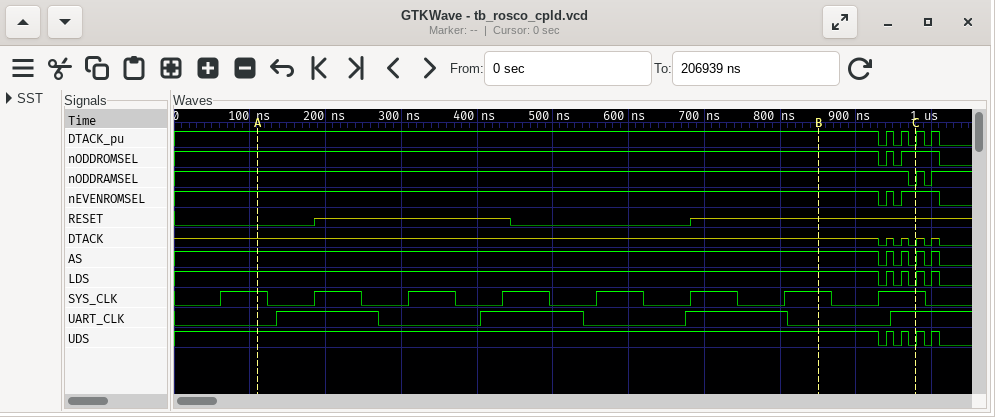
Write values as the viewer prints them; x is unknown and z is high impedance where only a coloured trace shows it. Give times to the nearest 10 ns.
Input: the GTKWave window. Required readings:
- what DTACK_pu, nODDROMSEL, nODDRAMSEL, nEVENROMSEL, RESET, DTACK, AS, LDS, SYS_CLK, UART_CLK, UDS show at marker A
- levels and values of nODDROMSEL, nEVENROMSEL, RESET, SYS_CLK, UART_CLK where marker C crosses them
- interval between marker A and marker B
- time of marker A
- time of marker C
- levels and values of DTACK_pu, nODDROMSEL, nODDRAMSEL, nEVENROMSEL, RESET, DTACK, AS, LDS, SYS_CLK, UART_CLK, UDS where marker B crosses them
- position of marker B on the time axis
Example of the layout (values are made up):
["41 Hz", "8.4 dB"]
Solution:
["DTACK_pu=1, nODDROMSEL=1, nODDRAMSEL=1, nEVENROMSEL=1, RESET=0, DTACK=z, AS=1, LDS=1, SYS_CLK=1, UART_CLK=0, UDS=1", "nODDROMSEL=1, nEVENROMSEL=1, RESET=z, SYS_CLK=1, UART_CLK=1", "740 ns", "110 ns", "980 ns", "DTACK_pu=1, nODDROMSEL=1, nODDRAMSEL=1, nEVENROMSEL=1, RESET=z, DTACK=z, AS=1, LDS=1, SYS_CLK=1, UART_CLK=0, UDS=1", "850 ns"]
